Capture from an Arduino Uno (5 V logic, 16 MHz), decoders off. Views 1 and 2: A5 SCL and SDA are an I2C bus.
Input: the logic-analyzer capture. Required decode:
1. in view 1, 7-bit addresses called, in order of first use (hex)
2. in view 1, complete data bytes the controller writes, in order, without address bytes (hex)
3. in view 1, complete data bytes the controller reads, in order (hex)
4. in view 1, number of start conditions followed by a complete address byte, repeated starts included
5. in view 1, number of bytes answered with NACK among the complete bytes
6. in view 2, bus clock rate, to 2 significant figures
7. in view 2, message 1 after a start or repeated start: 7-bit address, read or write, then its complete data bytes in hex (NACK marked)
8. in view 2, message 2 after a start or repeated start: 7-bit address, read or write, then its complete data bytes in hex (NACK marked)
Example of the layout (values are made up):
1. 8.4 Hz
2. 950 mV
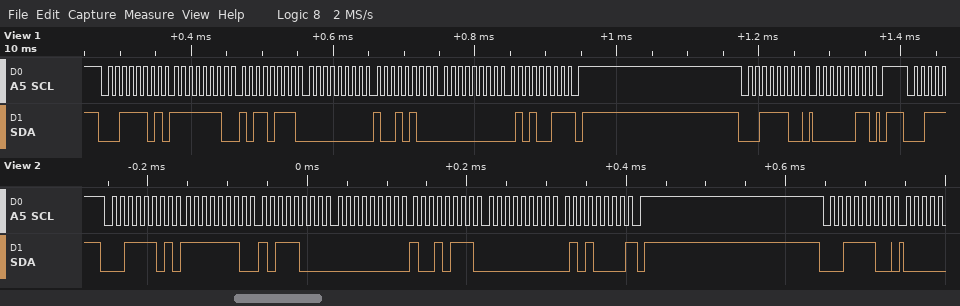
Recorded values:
1. 0x1E
2. 03
3. FE B7 00 94 00 53
4. 2
5. 1
6. 100 kHz
7. 0x1E read: FE B8 00 97 00 50 NACK
8. 0x1E write
